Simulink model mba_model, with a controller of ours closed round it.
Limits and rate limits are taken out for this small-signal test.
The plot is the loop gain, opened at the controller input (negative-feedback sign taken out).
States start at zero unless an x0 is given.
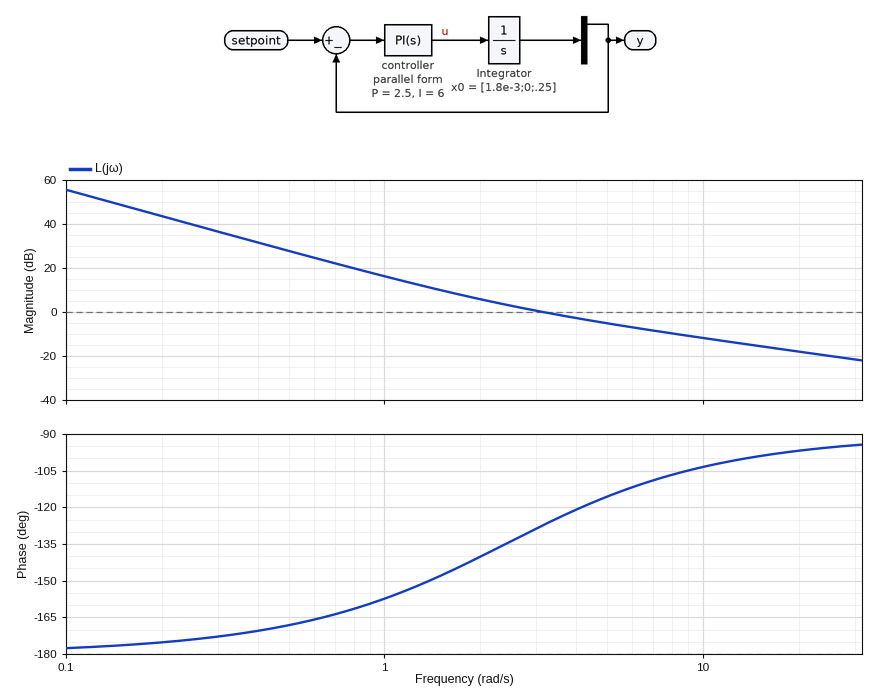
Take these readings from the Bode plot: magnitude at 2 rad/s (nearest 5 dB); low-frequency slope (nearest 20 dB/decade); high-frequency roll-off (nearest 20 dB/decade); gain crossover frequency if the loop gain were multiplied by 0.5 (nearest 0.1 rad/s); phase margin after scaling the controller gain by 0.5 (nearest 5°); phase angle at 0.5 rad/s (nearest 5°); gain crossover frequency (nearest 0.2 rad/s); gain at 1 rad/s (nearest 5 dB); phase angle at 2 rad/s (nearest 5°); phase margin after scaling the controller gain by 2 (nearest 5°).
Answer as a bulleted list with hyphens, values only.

- 5 dB
- -40 dB/decade
- -20 dB/decade
- 2.0 rad/s
- 40°
- -170°
- 3.2 rad/s
- 15 dB
- -140°
- 65°
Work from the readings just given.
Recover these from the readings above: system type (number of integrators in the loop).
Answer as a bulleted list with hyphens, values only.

- 2
